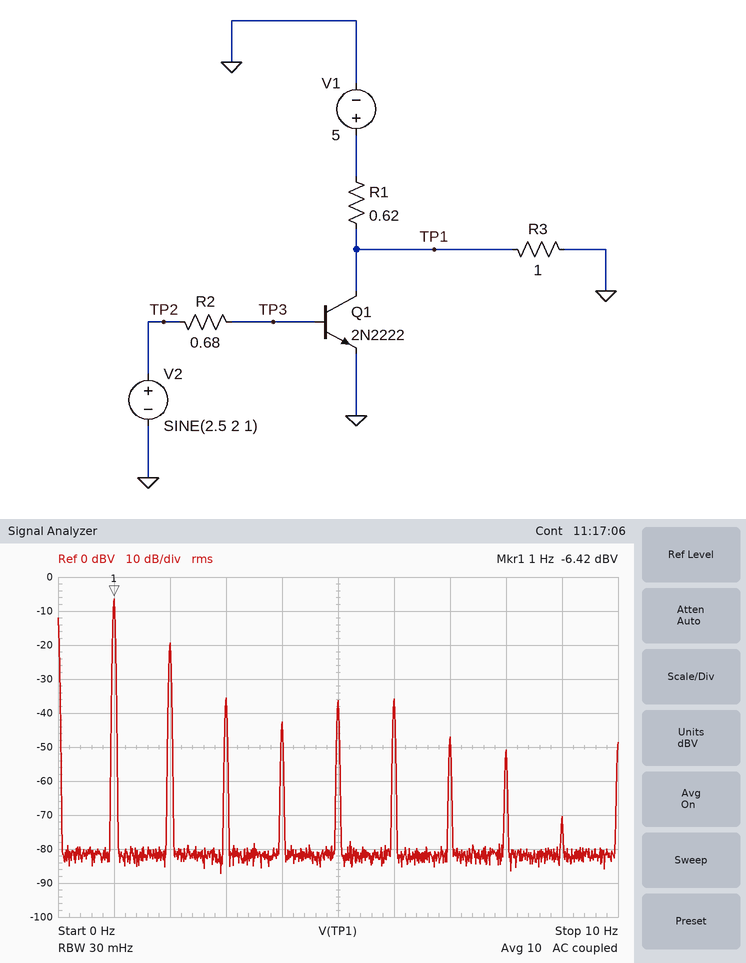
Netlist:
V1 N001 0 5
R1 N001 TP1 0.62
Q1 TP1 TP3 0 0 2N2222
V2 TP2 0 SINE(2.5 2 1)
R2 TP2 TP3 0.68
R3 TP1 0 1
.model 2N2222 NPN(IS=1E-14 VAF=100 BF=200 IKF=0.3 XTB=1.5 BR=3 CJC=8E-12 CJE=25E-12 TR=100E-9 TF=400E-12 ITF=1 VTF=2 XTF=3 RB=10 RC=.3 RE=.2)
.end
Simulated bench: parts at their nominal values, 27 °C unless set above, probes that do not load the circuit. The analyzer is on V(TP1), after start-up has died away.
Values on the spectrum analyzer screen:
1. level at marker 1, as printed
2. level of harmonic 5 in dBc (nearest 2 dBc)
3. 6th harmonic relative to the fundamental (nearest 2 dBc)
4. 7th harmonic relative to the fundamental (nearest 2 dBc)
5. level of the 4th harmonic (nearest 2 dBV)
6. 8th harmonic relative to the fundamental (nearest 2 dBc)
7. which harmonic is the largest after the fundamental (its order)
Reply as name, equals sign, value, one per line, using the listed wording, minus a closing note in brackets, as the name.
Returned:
level at marker 1, as printed = -6.42 dBV
level of harmonic 5 in dBc = -30 dBc
6th harmonic relative to the fundamental = -30 dBc
7th harmonic relative to the fundamental = -40 dBc
level of the 4th harmonic = -42 dBV
8th harmonic relative to the fundamental = -44 dBc
which harmonic is the largest after the fundamental = 2
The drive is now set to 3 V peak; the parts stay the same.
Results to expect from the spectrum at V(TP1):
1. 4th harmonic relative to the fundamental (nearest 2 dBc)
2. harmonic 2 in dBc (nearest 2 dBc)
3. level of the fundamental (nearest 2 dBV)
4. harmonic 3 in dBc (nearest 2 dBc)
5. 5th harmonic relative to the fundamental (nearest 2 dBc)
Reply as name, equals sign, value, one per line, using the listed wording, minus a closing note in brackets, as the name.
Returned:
4th harmonic relative to the fundamental = -20 dBc
harmonic 2 in dBc = -16 dBc
level of the fundamental = -6 dBV
harmonic 3 in dBc = -14 dBc
5th harmonic relative to the fundamental = -46 dBc
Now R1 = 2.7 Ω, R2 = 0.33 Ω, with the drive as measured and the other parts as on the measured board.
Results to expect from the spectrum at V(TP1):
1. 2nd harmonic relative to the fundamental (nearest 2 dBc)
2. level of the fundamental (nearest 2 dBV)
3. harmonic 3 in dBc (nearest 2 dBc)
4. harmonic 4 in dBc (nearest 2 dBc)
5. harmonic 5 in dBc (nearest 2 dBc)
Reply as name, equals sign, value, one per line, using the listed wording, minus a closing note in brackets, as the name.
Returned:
2nd harmonic relative to the fundamental = -2 dBc
level of the fundamental = -14 dBV
harmonic 3 in dBc = -8 dBc
harmonic 4 in dBc = -24 dBc
harmonic 5 in dBc = -18 dBc
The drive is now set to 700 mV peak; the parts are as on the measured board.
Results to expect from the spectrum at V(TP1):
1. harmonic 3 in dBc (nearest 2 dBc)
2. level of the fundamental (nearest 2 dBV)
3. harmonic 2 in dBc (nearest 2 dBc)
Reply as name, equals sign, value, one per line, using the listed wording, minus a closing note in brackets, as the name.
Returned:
harmonic 3 in dBc = -46 dBc
level of the fundamental = -16 dBV
harmonic 2 in dBc = -26 dBc
